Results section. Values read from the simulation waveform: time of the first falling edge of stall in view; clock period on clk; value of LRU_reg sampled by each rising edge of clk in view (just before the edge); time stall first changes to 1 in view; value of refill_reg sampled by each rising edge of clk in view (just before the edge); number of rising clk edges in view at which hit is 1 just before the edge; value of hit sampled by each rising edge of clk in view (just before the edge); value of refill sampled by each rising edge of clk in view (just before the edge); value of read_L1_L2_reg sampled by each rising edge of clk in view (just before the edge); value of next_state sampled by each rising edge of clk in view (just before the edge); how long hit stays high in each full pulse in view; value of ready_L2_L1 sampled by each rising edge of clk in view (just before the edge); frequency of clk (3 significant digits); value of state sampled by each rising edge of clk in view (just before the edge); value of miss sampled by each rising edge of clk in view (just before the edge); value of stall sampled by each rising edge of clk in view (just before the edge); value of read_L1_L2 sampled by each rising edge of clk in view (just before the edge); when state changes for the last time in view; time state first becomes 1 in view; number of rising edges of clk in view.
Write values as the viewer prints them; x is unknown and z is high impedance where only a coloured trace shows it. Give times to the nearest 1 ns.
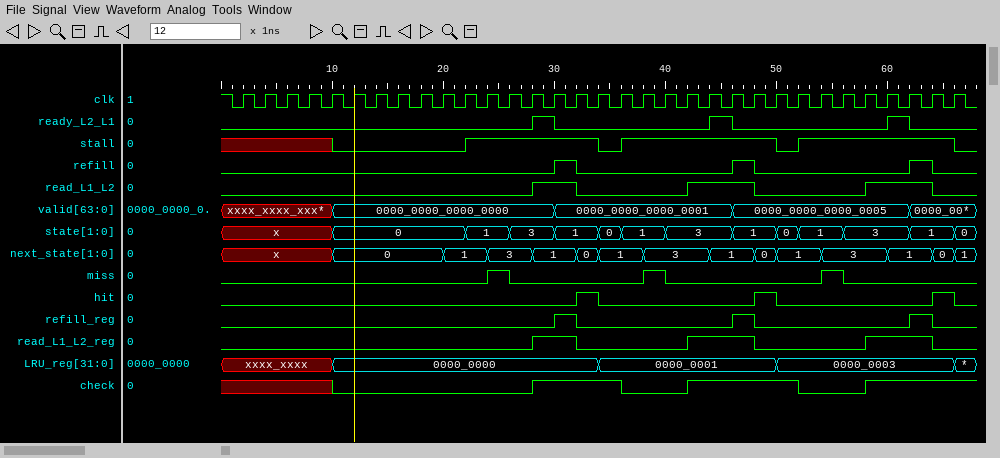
34 ns
2 ns
xxxx_xxxx, xxxx_xxxx, xxxx_xxxx, xxxx_xxxx, xxxx_xxxx, 0000_0000, 0000_0000, 0000_0000, 0000_0000, 0000_0000, 0000_0000, 0000_0000, 0000_0000, 0000_0000, 0000_0000, 0000_0000, 0000_0000, 0000_0001, 0000_0001, 0000_0001, 0000_0001, 0000_0001, 0000_0001, 0000_0001, 0000_0001, 0000_0003, 0000_0003, 0000_0003, 0000_0003, 0000_0003, 0000_0003, 0000_0003, 0000_0003
22 ns
0 0 0 0 0 0 0 0 0 0 0 0 0 0 0 1 0 0 0 0 0 0 0 1 0 0 0 0 0 0 0 1 0
3
0 0 0 0 0 0 0 0 0 0 0 0 0 0 0 0 1 0 0 0 0 0 0 0 1 0 0 0 0 0 0 0 1
0 0 0 0 0 0 0 0 0 0 0 0 0 0 0 1 0 0 0 0 0 0 0 1 0 0 0 0 0 0 0 1 0
0 0 0 0 0 0 0 0 0 0 0 0 0 0 1 1 0 0 0 0 0 1 1 1 0 0 0 0 0 1 1 1 0
x, x, x, x, x, 0, 0, 0, 0, 0, 1, 1, 3, 3, 1, 1, 0, 1, 1, 3, 3, 3, 1, 1, 0, 1, 1, 3, 3, 3, 1, 1, 0
2 ns, 2 ns, 2 ns
0 0 0 0 0 0 0 0 0 0 0 0 0 0 1 0 0 0 0 0 0 0 1 0 0 0 0 0 0 0 1 0 0
500 MHz
x, x, x, x, x, 0, 0, 0, 0, 0, 0, 1, 1, 3, 3, 1, 1, 0, 1, 1, 3, 3, 3, 1, 1, 0, 1, 1, 3, 3, 3, 1, 1
0 0 0 0 0 0 0 0 0 0 0 0 1 0 0 0 0 0 0 1 0 0 0 0 0 0 0 1 0 0 0 0 0
x x x x x 0 0 0 0 0 0 1 1 1 1 1 1 0 1 1 1 1 1 1 1 0 1 1 1 1 1 1 1
0 0 0 0 0 0 0 0 0 0 0 0 0 0 1 1 0 0 0 0 0 1 1 1 0 0 0 0 0 1 1 1 0
66 ns
22 ns
33
